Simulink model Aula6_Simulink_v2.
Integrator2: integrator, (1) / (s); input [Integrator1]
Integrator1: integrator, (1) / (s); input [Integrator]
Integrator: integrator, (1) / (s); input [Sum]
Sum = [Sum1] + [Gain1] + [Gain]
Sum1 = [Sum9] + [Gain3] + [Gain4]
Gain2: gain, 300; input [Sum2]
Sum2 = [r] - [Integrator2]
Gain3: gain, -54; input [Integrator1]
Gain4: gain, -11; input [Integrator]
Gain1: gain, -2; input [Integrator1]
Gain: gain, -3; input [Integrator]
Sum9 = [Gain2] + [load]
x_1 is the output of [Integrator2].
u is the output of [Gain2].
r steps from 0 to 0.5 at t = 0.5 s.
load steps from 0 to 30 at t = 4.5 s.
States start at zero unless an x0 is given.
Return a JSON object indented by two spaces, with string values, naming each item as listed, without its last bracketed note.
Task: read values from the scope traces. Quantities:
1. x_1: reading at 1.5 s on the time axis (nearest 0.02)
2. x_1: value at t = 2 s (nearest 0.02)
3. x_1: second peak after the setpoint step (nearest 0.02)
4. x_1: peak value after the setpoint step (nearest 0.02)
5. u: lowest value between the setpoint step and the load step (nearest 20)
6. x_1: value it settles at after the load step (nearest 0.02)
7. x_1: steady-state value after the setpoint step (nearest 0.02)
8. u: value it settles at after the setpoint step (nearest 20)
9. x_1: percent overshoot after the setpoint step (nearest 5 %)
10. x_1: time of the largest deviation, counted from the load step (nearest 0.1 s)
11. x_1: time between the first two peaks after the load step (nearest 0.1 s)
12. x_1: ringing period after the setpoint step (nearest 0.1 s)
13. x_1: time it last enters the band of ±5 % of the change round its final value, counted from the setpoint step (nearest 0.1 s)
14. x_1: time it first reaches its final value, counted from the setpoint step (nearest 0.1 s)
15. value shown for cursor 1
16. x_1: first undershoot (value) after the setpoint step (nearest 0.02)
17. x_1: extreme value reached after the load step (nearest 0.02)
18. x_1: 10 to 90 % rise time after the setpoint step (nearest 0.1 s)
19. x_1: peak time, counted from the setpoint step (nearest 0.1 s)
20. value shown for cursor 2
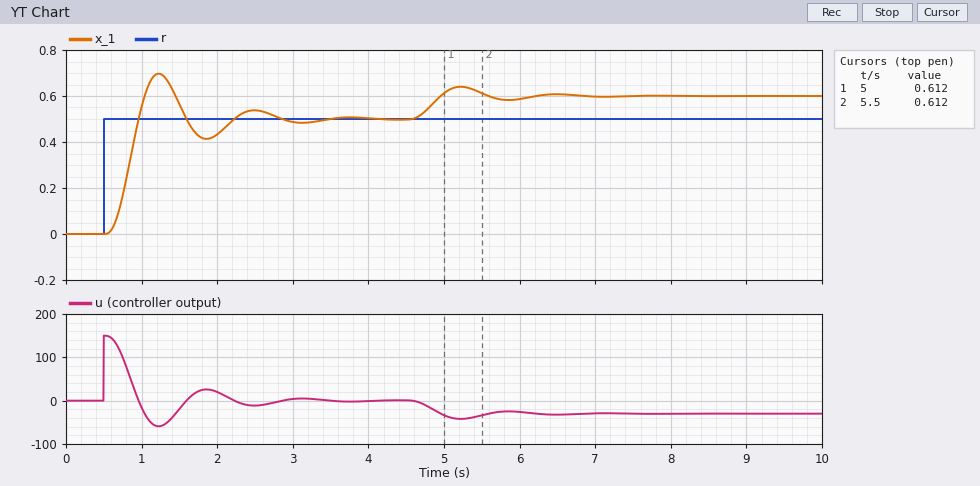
{
  "x_1: reading at 1.5 s on the time axis": "0.56",
  "x_1: value at t = 2 s": "0.44",
  "x_1: second peak after the setpoint step": "0.54",
  "x_1: peak value after the setpoint step": "0.70",
  "u: lowest value between the setpoint step and the load step": "-60",
  "x_1: value it settles at after the load step": "0.60",
  "x_1: steady-state value after the setpoint step": "0.50",
  "u: value it settles at after the setpoint step": "0",
  "x_1: percent overshoot after the setpoint step": "40 %",
  "x_1: time of the largest deviation, counted from the load step": "0.7 s",
  "x_1: time between the first two peaks after the load step": "1.3 s",
  "x_1: ringing period after the setpoint step": "1.3 s",
  "x_1: time it last enters the band of ±5 % of the change round its final value, counted from the setpoint step": "2.2 s",
  "x_1: time it first reaches its final value, counted from the setpoint step": "0.5 s",
  "value shown for cursor 1": "0.612",
  "x_1: first undershoot (value) after the setpoint step": "0.42",
  "x_1: extreme value reached after the load step": "0.64",
  "x_1: 10 to 90 % rise time after the setpoint step": "0.3 s",
  "x_1: peak time, counted from the setpoint step": "0.7 s",
  "value shown for cursor 2": "0.612"
}
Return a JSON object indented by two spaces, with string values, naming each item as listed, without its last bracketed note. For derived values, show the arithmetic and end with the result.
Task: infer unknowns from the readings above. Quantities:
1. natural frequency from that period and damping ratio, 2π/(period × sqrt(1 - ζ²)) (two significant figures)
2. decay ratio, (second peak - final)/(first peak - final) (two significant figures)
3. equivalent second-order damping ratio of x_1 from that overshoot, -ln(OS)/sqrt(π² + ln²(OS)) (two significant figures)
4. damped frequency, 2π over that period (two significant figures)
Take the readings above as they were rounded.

{
  "natural frequency from that period and damping ratio, 2π/(period × sqrt(1 - ζ²))": "2π / (1.3 × sqrt(1 - 0.28²)) = 5.0 rad/s",
  "decay ratio, (second peak - final)/(first peak - final)": "(0.54 - 0.5) / (0.7 - 0.5) = 0.20",
  "equivalent second-order damping ratio of x_1 from that overshoot, -ln(OS)/sqrt(π² + ln²(OS))": "ln(0.4) = -0.916; 0.916 / sqrt(9.870 + 0.840) = 0.28",
  "damped frequency, 2π over that period": "2π / 1.3 = 4.8 rad/s"
}
